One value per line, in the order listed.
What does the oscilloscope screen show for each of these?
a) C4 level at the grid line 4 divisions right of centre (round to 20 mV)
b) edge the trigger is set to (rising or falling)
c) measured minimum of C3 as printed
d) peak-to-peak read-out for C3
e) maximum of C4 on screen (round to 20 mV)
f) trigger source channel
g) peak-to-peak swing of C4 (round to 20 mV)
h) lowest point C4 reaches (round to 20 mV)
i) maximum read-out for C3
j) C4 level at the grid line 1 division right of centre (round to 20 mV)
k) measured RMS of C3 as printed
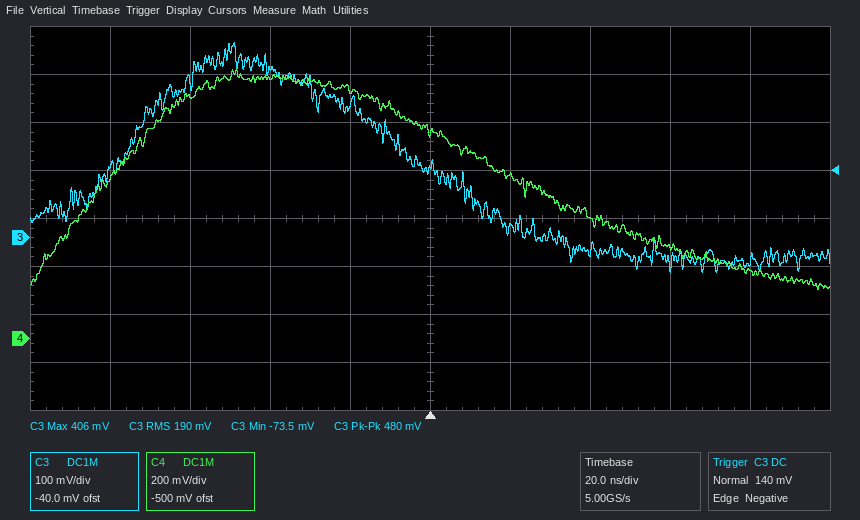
280 mV
falling
-73.5 mV
480 mV
1.12 V
C3
920 mV
200 mV
406 mV
680 mV
190 mV
